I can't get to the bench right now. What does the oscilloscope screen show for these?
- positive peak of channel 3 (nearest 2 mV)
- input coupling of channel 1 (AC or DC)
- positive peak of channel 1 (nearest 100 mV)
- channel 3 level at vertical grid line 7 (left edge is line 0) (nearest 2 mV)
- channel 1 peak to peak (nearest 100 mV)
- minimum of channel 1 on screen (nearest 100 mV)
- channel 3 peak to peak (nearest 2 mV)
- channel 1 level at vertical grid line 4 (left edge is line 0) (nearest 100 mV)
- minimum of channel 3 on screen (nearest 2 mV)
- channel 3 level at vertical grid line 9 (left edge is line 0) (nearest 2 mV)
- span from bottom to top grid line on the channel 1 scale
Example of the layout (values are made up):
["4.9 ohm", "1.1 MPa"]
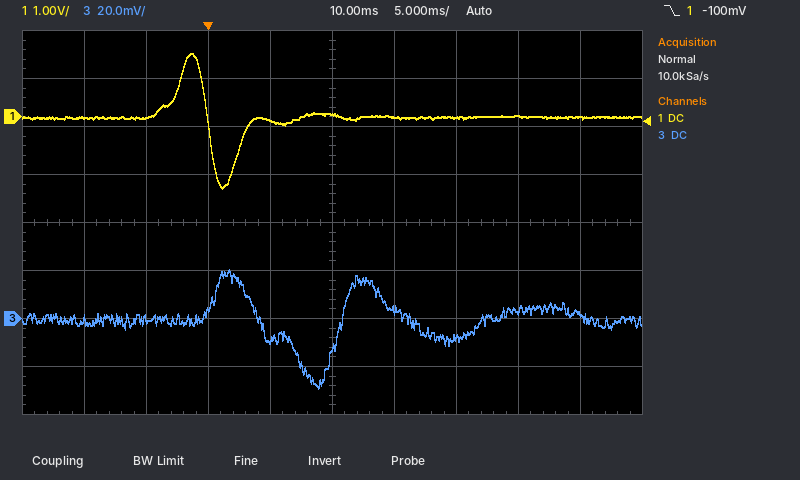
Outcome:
["20 mV", "DC", "1.3 V", "-8 mV", "2.8 V", "-1.5 V", "50 mV", "-100 mV", "-30 mV", "2 mV", "8 V"]
